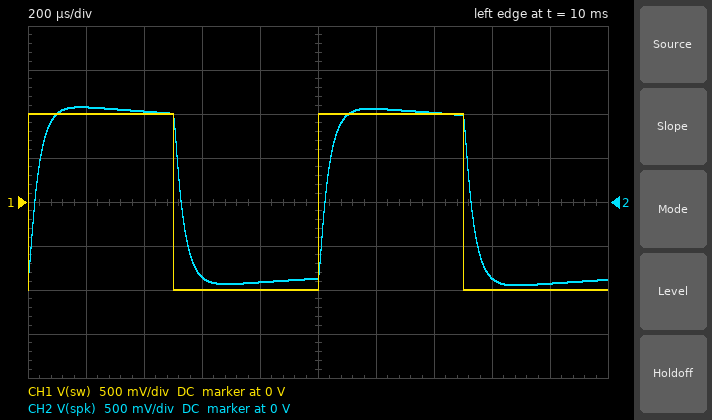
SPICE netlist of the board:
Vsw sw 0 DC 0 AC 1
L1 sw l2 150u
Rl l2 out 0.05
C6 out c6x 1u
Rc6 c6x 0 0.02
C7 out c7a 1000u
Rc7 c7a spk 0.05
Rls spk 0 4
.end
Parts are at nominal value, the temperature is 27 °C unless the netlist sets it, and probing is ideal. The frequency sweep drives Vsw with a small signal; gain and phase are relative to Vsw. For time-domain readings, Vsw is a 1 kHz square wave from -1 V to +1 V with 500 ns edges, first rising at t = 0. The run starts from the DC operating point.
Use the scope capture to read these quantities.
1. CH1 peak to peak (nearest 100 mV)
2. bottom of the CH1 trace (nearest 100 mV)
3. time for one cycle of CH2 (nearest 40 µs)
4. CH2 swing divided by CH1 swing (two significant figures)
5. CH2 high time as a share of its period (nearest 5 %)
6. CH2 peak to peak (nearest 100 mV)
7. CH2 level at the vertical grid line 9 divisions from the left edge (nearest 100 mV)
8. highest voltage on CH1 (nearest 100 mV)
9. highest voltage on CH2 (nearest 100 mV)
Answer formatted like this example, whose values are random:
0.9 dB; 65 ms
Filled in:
2.0 V; -1.0 V; 1.00 ms; 1.0; 50 %; 2.0 V; -900 mV; 1.0 V; 1.1 V
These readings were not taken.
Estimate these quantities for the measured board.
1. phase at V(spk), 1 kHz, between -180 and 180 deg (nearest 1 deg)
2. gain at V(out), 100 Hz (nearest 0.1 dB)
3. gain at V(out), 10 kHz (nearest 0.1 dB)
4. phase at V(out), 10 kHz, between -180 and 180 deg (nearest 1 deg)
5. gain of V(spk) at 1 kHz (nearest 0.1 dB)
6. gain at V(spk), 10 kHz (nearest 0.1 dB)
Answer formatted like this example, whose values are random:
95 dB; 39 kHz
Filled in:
-11 deg; 0 dB; -7.5 dB; -80 deg; -0.3 dB; -7.6 dB
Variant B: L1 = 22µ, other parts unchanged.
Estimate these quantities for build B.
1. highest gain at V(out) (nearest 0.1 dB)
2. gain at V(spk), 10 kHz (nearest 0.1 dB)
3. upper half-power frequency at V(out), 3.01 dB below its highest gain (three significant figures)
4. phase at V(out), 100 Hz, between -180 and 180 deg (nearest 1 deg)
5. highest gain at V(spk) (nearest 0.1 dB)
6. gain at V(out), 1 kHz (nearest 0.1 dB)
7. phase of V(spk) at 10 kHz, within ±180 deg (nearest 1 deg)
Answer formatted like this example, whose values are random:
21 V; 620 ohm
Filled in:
0.4 dB; 0 dB; 38.3 kHz; 0 deg; 0.3 dB; -0.1 dB; -20 deg
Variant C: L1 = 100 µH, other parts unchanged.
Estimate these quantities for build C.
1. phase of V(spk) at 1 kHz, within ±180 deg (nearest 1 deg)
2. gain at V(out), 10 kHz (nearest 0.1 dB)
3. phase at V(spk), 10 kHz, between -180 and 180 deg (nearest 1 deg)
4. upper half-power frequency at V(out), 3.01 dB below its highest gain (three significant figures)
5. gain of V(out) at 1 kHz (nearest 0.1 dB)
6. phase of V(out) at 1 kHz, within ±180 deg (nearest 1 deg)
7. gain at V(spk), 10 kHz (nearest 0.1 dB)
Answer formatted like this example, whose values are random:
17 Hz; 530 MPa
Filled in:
-7 deg; -4.5 dB; -68 deg; 7.59 kHz; -0.1 dB; -9 deg; -4.6 dB
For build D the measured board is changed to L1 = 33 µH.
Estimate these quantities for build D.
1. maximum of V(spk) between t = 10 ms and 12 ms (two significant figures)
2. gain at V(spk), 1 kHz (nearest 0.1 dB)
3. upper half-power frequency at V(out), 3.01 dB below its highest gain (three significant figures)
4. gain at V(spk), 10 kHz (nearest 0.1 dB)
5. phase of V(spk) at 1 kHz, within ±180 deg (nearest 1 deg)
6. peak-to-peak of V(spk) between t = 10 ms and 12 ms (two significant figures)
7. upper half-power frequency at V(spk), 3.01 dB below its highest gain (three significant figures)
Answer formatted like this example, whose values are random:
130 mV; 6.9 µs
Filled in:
1.2 V; -0.2 dB; 27.4 kHz; -0.3 dB; -1 deg; 2.3 V; 27.7 kHz
